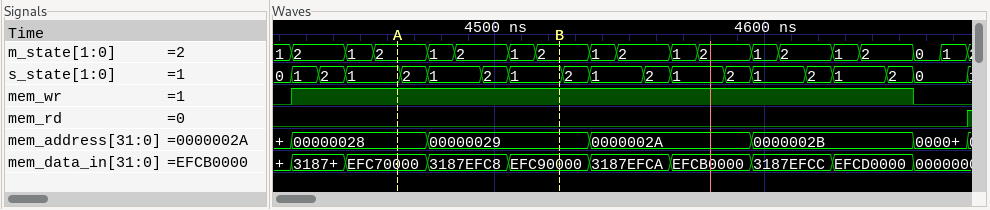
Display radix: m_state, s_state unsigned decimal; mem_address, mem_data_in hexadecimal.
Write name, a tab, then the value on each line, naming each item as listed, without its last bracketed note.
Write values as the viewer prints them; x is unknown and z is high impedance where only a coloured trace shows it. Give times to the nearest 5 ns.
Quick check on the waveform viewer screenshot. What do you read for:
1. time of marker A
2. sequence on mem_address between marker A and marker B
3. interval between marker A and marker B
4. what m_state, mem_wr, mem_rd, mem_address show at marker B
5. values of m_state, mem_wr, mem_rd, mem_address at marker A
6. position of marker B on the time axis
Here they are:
time of marker A	4465 ns
sequence on mem_address between marker A and marker B	00000028, 00000029
interval between marker A and marker B	60 ns
what m_state, mem_wr, mem_rd, mem_address show at marker B	m_state=2, mem_wr=1, mem_rd=0, mem_address=00000029
values of m_state, mem_wr, mem_rd, mem_address at marker A	m_state=2, mem_wr=1, mem_rd=0, mem_address=00000028
position of marker B on the time axis	4525 ns
